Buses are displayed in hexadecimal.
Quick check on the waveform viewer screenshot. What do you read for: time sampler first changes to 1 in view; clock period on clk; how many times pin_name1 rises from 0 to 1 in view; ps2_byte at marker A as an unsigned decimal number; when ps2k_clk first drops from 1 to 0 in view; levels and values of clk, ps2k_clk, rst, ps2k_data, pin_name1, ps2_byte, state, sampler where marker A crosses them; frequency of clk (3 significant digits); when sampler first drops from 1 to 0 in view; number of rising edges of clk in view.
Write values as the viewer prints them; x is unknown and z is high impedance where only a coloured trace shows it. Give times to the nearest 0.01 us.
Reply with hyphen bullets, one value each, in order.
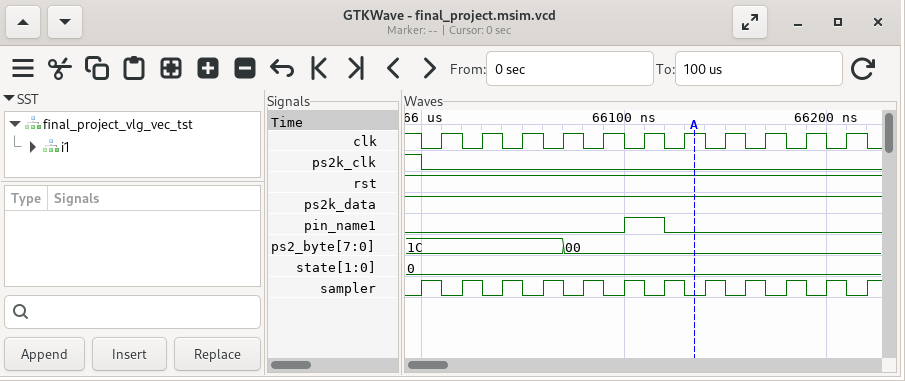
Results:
- 66 us
- 0.02 us
- 1
- 0
- 66 us
- clk=1, ps2k_clk=0, rst=1, ps2k_data=1, pin_name1=0, ps2_byte=00, state=0, sampler=0
- 50.0 MHz
- 66.01 us
- 11
